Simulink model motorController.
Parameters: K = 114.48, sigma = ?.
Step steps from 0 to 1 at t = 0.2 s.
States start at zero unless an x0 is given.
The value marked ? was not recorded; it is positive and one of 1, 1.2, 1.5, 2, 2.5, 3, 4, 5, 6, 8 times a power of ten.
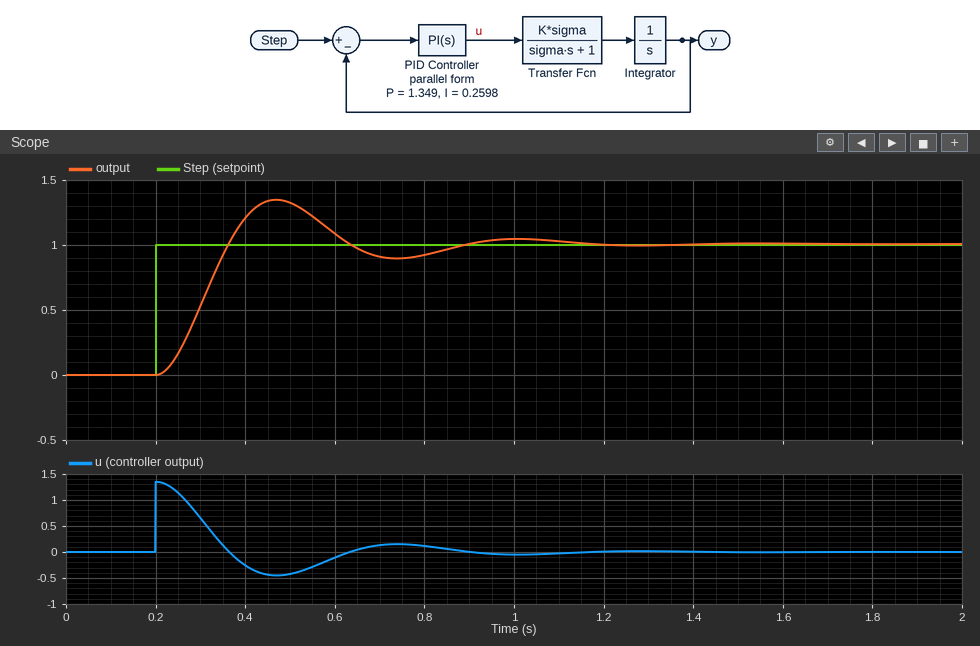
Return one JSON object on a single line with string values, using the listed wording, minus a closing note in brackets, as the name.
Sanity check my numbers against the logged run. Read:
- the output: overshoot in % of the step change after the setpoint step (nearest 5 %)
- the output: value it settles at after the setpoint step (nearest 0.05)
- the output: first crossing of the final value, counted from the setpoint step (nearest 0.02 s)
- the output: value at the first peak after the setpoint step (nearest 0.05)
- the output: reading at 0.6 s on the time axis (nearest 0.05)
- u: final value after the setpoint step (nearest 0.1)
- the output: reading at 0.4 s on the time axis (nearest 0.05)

{"the output: overshoot in % of the step change after the setpoint step": "35 %", "the output: value it settles at after the setpoint step": "1.00", "the output: first crossing of the final value, counted from the setpoint step": "0.16 s", "the output: value at the first peak after the setpoint step": "1.35", "the output: reading at 0.6 s on the time axis": "1.10", "u: final value after the setpoint step": "0.0", "the output: reading at 0.4 s on the time axis": "1.20"}
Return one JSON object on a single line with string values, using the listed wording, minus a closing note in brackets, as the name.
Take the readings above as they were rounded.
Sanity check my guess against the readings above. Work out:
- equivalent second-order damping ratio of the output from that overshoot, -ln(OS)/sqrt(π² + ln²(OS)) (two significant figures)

{"equivalent second-order damping ratio of the output from that overshoot, -ln(OS)/sqrt(π² + ln²(OS))": "0.32"}
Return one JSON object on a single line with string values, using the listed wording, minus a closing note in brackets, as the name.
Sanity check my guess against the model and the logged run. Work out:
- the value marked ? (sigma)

{"the value marked ?": "0.12"}
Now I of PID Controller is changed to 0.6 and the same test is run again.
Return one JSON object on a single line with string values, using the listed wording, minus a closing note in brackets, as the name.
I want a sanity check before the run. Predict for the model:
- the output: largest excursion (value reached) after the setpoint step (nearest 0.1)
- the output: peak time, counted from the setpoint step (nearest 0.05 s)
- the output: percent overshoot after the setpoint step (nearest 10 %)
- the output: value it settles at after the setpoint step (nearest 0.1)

{"the output: largest excursion (value reached) after the setpoint step": "1.4", "the output: peak time, counted from the setpoint step": "0.25 s", "the output: percent overshoot after the setpoint step": "40 %", "the output: value it settles at after the setpoint step": "1.0"}
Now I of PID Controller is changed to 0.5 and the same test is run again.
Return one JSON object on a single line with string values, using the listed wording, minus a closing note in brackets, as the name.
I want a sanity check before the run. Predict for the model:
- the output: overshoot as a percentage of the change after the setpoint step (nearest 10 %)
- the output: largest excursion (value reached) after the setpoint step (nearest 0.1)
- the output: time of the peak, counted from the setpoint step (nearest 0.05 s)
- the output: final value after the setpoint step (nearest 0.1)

{"the output: overshoot as a percentage of the change after the setpoint step": "40 %", "the output: largest excursion (value reached) after the setpoint step": "1.4", "the output: time of the peak, counted from the setpoint step": "0.25 s", "the output: final value after the setpoint step": "1.0"}
